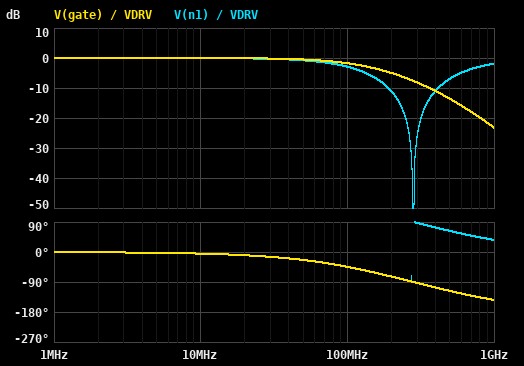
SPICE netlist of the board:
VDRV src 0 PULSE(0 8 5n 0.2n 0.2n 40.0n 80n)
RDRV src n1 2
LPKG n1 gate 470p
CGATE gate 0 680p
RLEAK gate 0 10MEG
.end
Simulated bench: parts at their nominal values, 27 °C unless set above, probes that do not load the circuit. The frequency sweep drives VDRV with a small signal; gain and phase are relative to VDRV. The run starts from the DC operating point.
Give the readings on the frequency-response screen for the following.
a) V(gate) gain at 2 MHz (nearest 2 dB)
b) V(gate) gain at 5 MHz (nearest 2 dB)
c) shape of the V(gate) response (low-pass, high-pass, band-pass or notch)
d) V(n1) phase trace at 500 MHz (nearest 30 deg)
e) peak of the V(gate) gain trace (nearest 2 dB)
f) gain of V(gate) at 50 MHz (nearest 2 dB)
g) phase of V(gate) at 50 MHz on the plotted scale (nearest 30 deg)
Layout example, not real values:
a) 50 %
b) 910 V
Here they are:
a) 0 dB
b) 0 dB
c) low-pass
d) 60 deg
e) 0 dB
f) 0 dB
g) -30 deg
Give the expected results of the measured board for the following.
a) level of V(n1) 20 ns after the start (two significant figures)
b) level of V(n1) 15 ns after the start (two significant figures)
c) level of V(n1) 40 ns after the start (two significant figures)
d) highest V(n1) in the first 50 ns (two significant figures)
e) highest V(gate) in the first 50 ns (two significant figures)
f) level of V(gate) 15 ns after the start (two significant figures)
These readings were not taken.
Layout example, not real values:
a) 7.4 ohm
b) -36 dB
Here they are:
a) 8.0 V
b) 8.0 V
c) 8.0 V
d) 8.0 V
e) 8.0 V
f) 8.0 V
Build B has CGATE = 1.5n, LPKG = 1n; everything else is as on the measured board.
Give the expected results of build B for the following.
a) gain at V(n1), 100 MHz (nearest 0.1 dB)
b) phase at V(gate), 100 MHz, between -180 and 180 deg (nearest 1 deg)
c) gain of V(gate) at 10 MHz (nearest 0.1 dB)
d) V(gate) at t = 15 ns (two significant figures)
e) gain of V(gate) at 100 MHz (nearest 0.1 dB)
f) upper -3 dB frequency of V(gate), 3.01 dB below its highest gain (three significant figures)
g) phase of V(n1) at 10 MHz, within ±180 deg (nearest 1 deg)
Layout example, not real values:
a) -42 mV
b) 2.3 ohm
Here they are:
a) -13.5 dB
b) -78 deg
c) -0.1 dB
d) 7.8 V
e) -5.7 dB
f) 63.1 MHz
g) -11 deg
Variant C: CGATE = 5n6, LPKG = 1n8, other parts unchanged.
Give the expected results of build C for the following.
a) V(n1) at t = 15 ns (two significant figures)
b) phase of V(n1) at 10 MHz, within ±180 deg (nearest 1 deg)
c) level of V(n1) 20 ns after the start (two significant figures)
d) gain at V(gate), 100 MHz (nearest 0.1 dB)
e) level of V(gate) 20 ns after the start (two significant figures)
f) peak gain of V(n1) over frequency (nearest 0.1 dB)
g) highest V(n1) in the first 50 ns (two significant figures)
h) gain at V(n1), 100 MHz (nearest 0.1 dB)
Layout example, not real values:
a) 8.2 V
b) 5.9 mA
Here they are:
a) 4.3 V
b) -36 deg
c) 5.7 V
d) -17.7 dB
e) 5.9 V
f) 0 dB
g) 7.8 V
h) -8.2 dB
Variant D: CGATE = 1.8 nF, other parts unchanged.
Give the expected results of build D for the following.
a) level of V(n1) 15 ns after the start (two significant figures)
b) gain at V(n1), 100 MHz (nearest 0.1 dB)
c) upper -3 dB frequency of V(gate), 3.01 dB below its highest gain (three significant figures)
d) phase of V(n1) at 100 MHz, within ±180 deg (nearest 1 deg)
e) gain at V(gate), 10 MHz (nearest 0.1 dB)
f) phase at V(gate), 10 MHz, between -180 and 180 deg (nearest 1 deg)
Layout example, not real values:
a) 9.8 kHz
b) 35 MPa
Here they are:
a) 7.5 V
b) -11.0 dB
c) 47.3 MHz
d) -74 deg
e) -0.2 dB
f) -13 deg
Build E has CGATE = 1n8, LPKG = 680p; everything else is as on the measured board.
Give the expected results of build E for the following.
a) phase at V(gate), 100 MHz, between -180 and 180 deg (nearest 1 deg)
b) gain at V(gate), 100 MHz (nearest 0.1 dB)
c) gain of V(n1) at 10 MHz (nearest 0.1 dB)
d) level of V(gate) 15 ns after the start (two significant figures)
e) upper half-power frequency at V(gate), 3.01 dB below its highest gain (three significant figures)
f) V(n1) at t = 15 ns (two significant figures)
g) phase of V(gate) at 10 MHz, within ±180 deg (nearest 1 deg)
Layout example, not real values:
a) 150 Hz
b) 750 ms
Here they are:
a) -77 deg
b) -7.3 dB
c) -0.2 dB
d) 7.6 V
e) 48.8 MHz
f) 7.5 V
g) -13 deg
